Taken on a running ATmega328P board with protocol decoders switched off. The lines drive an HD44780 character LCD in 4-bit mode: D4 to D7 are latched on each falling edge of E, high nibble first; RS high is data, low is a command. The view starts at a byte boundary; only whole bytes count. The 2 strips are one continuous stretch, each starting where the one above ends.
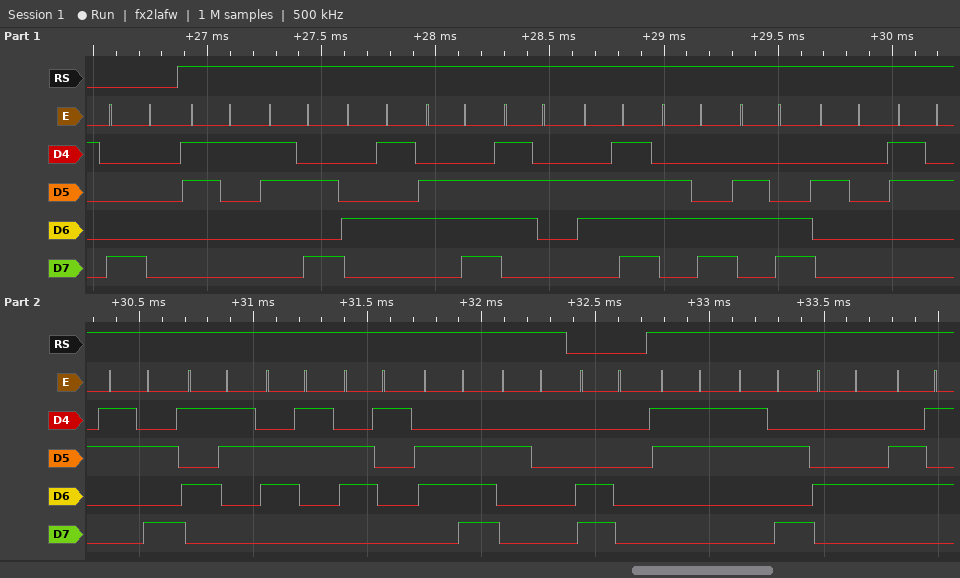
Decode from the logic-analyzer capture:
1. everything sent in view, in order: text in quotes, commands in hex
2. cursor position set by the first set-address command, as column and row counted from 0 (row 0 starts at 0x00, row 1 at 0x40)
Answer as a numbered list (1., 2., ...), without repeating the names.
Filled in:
1. 0x80 "1:Enroll 2:Scan " 0xC0 "3:De"
2. column 0, row 0
